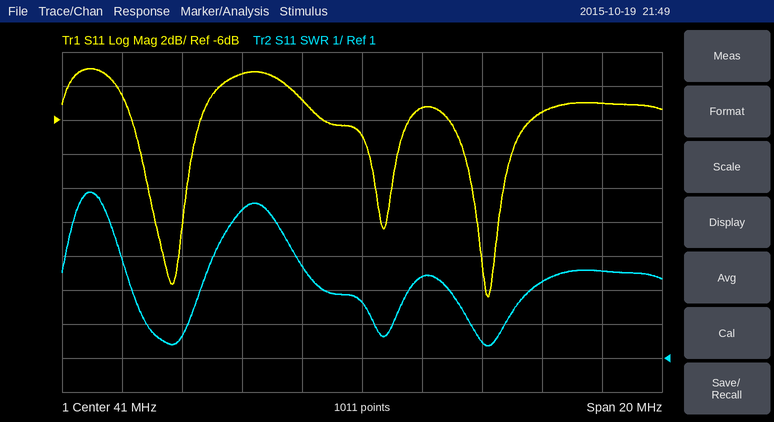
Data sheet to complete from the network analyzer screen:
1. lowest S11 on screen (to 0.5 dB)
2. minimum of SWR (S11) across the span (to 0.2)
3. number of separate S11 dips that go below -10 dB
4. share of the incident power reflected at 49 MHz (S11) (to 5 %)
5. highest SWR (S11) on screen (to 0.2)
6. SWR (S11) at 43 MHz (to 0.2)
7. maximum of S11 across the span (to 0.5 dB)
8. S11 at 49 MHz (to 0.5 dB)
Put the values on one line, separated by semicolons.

-16.5 dB; 1.4; 3; 30 %; 5.8; 3.4; -3.0 dB; -5.0 dB
